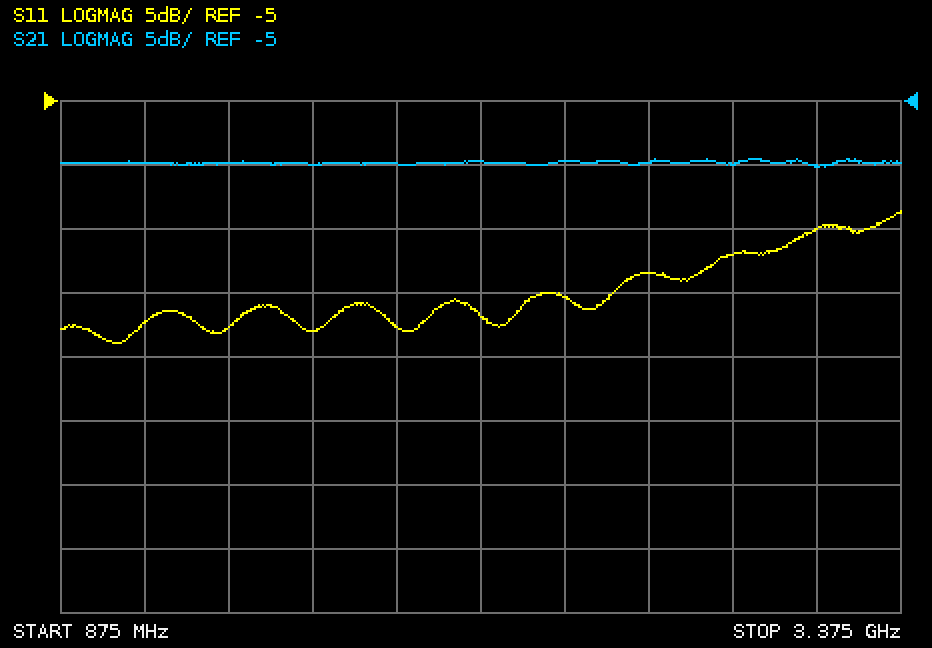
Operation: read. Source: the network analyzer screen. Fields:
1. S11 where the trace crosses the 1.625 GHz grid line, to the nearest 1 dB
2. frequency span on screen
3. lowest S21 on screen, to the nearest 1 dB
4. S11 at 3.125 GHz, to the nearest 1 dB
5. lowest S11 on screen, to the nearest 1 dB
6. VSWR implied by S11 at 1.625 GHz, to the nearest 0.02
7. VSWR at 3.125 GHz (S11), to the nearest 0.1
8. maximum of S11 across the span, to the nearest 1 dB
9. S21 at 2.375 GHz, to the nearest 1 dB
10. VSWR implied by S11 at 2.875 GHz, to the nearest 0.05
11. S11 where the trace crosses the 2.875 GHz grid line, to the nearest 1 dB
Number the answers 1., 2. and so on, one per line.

1. -23 dB
2. 2.5 GHz
3. -10 dB
4. -15 dB
5. -24 dB
6. 1.16
7. 1.4
8. -14 dB
9. -10 dB
10. 1.35
11. -17 dB
